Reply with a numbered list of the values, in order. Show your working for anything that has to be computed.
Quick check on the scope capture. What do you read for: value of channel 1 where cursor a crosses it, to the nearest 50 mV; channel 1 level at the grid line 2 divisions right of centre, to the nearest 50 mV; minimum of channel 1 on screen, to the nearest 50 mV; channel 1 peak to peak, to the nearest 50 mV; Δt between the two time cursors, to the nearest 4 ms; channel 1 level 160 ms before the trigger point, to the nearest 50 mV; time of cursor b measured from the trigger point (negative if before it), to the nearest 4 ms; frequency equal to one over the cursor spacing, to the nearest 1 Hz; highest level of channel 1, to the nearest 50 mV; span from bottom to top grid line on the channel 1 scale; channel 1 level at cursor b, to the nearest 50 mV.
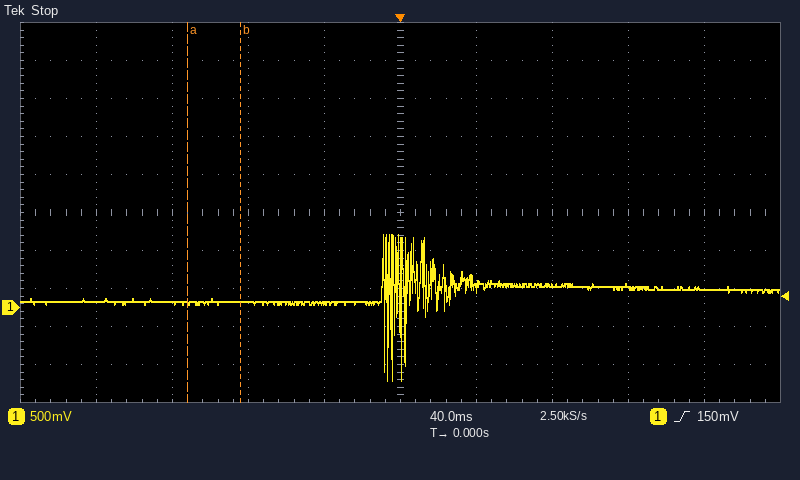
1. 50 mV
2. 300 mV
3. -950 mV
4. 950 mV − (-950 mV) = 1.90 V
5. 28 ms
6. 100 mV
7. -84 ms
8. 1 / 28 ms ≈ 36 Hz
9. 950 mV
10. 5 V
11. 100 mV
